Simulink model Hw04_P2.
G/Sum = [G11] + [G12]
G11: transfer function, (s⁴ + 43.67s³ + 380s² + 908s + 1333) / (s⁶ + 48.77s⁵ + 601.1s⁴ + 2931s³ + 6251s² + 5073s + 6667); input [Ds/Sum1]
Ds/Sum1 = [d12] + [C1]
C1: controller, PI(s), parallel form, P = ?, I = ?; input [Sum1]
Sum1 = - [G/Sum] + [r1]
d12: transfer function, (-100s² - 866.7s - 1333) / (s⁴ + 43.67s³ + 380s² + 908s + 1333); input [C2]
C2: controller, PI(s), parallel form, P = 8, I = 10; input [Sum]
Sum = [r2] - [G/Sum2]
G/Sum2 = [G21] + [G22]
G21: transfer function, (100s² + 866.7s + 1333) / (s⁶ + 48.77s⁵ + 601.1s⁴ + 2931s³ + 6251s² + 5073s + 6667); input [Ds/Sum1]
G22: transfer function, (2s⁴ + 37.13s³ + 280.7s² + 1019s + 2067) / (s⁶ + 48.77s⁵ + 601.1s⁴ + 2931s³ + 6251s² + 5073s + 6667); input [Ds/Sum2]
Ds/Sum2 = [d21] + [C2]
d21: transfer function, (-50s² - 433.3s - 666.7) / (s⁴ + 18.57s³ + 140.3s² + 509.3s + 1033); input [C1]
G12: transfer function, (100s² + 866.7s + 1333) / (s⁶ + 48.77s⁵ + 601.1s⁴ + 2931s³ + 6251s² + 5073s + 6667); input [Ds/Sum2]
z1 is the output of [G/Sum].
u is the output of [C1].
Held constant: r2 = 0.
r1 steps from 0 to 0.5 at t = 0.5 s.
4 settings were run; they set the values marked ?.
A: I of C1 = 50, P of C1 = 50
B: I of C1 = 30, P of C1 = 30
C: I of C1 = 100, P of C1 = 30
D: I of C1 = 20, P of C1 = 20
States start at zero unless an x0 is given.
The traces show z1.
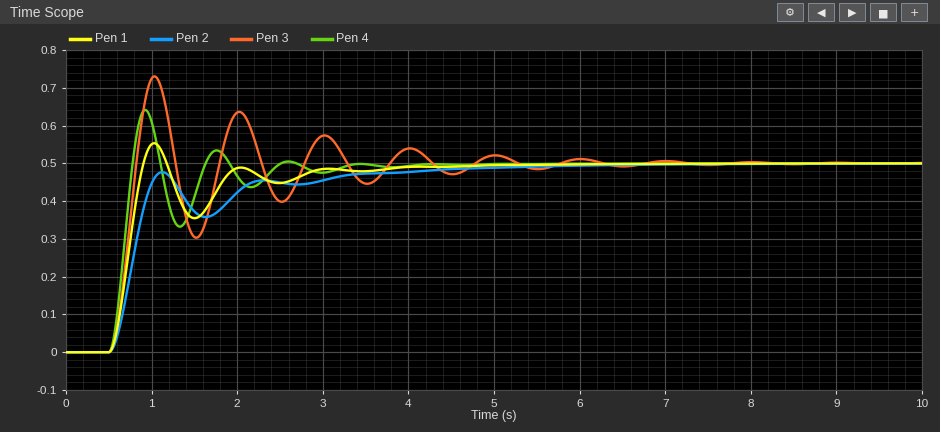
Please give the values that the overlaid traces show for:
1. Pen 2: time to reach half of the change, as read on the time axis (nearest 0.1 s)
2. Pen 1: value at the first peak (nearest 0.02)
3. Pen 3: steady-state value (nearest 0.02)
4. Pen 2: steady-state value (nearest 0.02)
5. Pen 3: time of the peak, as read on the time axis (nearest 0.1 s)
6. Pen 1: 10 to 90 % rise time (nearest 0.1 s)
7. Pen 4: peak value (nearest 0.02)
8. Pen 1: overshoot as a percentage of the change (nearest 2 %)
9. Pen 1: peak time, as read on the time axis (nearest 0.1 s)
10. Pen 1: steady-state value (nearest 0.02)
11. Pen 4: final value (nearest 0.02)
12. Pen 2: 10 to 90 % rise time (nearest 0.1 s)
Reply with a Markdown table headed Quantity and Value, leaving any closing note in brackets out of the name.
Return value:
| Quantity | Value |
|---|---|
| Pen 2: time to reach half of the change, as read on the time axis | 0.8 s |
| Pen 1: value at the first peak | 0.56 |
| Pen 3: steady-state value | 0.50 |
| Pen 2: steady-state value | 0.50 |
| Pen 3: time of the peak, as read on the time axis | 1.0 s |
| Pen 1: 10 to 90 % rise time | 0.3 s |
| Pen 4: peak value | 0.64 |
| Pen 1: overshoot as a percentage of the change | 10 % |
| Pen 1: peak time, as read on the time axis | 1.0 s |
| Pen 1: steady-state value | 0.50 |
| Pen 4: final value | 0.50 |
| Pen 2: 10 to 90 % rise time | 0.4 s |
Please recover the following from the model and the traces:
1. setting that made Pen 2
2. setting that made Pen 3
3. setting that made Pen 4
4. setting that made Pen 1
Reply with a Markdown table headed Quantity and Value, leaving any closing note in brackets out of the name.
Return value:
| Quantity | Value |
|---|---|
| setting that made Pen 2 | D |
| setting that made Pen 3 | C |
| setting that made Pen 4 | A |
| setting that made Pen 1 | B |
